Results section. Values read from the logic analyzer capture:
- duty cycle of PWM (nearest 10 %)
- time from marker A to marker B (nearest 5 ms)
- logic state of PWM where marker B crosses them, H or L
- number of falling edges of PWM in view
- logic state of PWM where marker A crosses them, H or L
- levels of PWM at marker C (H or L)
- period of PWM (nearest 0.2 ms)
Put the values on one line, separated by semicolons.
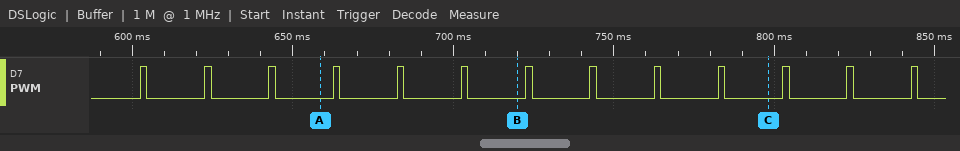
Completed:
10 %; 60 ms; PWM=L; 13; PWM=L; PWM=L; 20 ms
